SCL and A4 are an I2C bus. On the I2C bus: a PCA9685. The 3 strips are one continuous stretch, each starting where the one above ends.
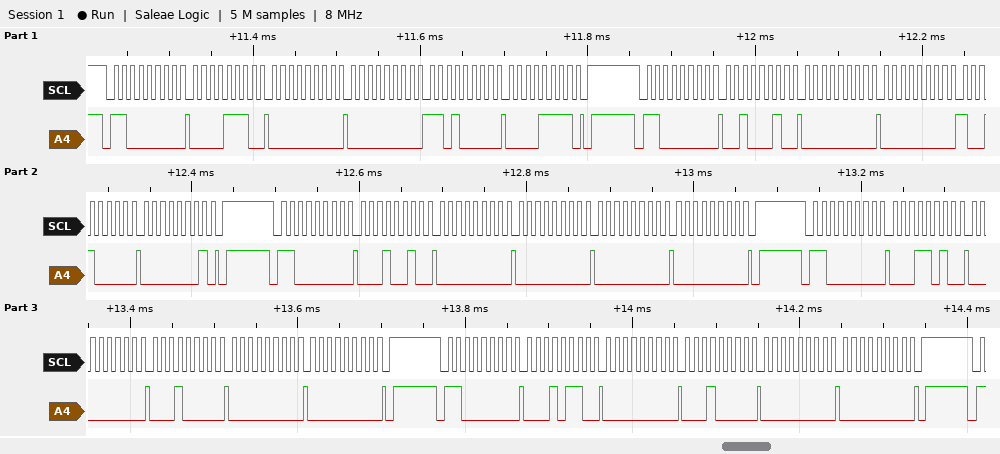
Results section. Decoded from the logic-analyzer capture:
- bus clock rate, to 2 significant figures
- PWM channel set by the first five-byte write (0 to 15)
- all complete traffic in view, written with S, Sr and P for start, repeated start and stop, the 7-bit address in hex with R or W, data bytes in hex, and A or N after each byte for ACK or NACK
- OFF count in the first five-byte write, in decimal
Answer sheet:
100 kHz
2
S 60W A 0E A 00 A 00 A D0 A 0F A P S 60W A 22 A 00 A 00 A 90 A 01 A P S 60W A 12 A 00 A 00 A 00 A 00 A P S 60W A 1A A 00 A 10 A 00 A 00 A P S 60W A 16 A 00 A 10 A 00 A 00 A P
4048
